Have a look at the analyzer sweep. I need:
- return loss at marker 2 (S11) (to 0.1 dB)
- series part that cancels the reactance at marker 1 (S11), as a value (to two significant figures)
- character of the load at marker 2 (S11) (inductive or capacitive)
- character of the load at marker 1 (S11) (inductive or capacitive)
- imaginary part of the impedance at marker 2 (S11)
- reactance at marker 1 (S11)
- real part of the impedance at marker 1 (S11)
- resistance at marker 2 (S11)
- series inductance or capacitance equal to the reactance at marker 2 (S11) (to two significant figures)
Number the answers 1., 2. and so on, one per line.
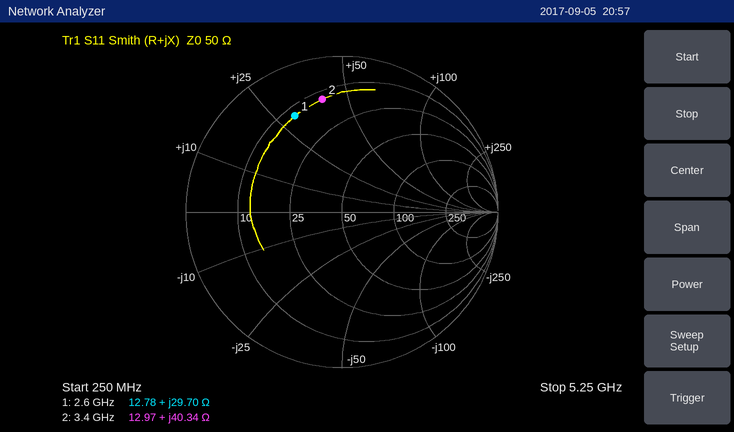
1. 2.7 dB
2. 2.1 pF
3. inductive
4. inductive
5. +40.34 Ω
6. +29.70 Ω
7. 12.78 Ω
8. 12.97 Ω
9. 1.9 nH
